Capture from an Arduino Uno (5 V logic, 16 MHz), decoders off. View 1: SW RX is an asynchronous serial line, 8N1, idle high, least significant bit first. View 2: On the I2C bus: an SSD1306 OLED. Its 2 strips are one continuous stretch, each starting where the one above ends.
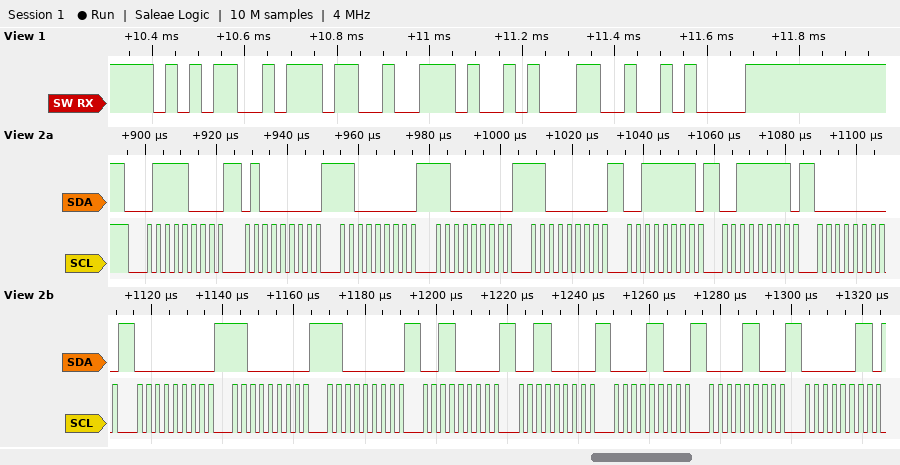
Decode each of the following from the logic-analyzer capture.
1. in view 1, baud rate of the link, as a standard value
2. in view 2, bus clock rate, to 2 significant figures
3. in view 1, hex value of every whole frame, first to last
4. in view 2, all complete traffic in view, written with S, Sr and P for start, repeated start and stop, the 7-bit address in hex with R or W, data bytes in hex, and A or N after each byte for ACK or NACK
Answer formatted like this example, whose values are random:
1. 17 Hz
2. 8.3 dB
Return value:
1. 38400 baud
2. 400 kHz
3. 35 37 2E 31 0A
4. S 3CW A 40 A C0 A C0 A C0 A 3F A 3F A 00 A 00 A C0 A C0 A 30 A 30 A 0C A 0C A 03 A
